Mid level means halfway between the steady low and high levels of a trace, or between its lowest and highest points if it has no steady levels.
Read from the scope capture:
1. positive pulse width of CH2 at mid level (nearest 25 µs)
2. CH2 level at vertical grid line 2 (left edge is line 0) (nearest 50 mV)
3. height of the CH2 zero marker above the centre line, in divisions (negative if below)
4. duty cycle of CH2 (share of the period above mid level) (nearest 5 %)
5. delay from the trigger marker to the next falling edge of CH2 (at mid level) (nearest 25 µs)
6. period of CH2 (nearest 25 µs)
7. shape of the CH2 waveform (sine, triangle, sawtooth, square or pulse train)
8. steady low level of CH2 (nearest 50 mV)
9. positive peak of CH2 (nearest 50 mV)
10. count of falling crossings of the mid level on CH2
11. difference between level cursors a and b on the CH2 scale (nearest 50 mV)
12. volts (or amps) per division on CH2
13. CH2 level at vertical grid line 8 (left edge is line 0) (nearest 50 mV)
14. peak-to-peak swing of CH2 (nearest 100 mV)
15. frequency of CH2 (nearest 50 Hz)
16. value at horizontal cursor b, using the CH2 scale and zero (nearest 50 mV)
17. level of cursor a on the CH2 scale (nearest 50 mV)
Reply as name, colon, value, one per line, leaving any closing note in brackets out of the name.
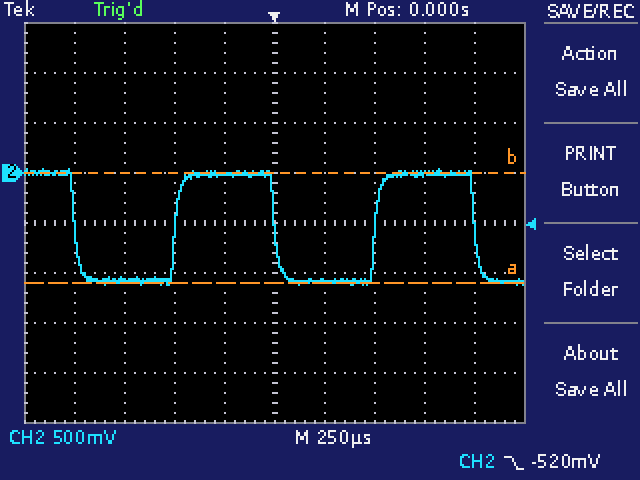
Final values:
positive pulse width of CH2 at mid level: 500 µs
CH2 level at vertical grid line 2 (left edge is line 0): -1.05 V
height of the CH2 zero marker above the centre line, in divisions: +1.0 div
duty cycle of CH2 (share of the period above mid level): 50 %
delay from the trigger marker to the next falling edge of CH2 (at mid level): 1.000 ms
period of CH2: 1.000 ms
shape of the CH2 waveform: square
steady low level of CH2: -1.10 V
positive peak of CH2: 50 mV
count of falling crossings of the mid level on CH2: 3
difference between level cursors a and b on the CH2 scale: 1.10 V
volts (or amps) per division on CH2: 500 mV
CH2 level at vertical grid line 8 (left edge is line 0): 0 mV
peak-to-peak swing of CH2: 1.20 V
frequency of CH2: 1.00 kHz
value at horizontal cursor b, using the CH2 scale and zero: 0 mV
level of cursor a on the CH2 scale: -1.10 V
